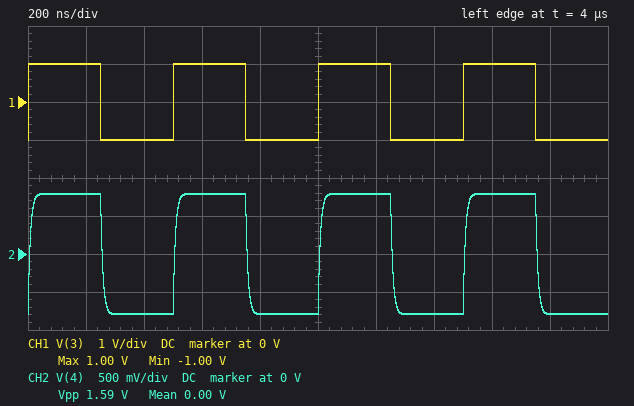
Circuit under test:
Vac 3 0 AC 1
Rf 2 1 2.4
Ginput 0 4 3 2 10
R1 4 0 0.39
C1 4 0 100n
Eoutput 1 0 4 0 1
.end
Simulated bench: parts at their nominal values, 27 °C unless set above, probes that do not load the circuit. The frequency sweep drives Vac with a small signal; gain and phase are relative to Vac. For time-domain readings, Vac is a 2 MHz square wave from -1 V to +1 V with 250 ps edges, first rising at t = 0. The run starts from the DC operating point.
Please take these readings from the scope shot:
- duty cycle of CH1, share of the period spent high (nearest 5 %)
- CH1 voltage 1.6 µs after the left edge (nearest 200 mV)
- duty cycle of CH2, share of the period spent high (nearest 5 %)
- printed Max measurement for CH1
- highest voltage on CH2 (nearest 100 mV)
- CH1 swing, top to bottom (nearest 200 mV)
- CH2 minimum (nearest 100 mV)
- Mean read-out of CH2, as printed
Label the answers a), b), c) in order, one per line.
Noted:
a) 50 %
b) 1.0 V
c) 50 %
d) 1.00 V
e) 800 mV
f) 2.0 V
g) -800 mV
h) 0.00 V
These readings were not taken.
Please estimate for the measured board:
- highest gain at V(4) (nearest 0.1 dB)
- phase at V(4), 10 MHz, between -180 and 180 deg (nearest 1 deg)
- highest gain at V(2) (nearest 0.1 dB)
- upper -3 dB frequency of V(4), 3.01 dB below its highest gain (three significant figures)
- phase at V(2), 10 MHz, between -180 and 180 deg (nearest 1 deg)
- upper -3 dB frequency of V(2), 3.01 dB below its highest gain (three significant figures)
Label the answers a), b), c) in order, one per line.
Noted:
a) -2.0 dB
b) -27 deg
c) -2.0 dB
d) 20.0 MHz
e) -27 deg
f) 20.0 MHz
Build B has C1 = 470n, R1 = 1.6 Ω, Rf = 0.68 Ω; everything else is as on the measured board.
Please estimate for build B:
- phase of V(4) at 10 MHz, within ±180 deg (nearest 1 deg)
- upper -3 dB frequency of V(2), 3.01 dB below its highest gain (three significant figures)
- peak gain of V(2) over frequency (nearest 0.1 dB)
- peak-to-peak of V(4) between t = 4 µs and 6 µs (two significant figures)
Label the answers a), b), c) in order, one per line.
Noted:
a) -70 deg
b) 3.60 MHz
c) -0.5 dB
d) 1.9 V
